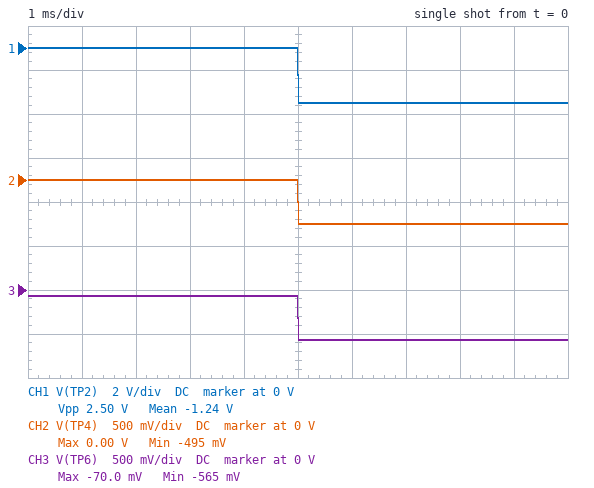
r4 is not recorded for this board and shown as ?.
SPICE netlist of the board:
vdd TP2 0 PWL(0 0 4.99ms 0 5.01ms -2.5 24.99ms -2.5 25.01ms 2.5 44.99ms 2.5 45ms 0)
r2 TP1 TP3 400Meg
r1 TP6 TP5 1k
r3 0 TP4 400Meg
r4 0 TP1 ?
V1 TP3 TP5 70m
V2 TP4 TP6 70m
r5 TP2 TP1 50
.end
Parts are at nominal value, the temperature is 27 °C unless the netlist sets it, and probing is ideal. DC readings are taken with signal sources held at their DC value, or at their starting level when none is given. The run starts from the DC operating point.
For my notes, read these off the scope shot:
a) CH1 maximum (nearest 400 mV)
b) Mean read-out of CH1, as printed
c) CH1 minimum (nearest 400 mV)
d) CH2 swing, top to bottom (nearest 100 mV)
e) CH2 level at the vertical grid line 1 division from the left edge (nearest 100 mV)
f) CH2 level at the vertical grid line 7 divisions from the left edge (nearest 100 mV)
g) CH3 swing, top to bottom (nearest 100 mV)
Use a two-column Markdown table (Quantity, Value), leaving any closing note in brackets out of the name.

| Quantity | Value |
|---|---|
| CH1 maximum | 0 V |
| Mean read-out of CH1, as printed | -1.24 V |
| CH1 minimum | -2.4 V |
| CH2 swing, top to bottom | 500 mV |
| CH2 level at the vertical grid line 1 division from the left edge | 0 V |
| CH2 level at the vertical grid line 7 divisions from the left edge | -500 mV |
| CH3 swing, top to bottom | 500 mV |
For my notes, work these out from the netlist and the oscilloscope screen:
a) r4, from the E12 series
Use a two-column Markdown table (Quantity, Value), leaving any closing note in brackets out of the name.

| Quantity | Value |
|---|---|
| r4, from the E12 series | 33 Ω |
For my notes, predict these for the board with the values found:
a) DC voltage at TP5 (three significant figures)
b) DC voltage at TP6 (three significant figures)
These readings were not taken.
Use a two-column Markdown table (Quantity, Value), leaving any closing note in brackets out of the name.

| Quantity | Value |
|---|---|
| DC voltage at TP5 | -70.0 mV |
| DC voltage at TP6 | -70.0 mV |
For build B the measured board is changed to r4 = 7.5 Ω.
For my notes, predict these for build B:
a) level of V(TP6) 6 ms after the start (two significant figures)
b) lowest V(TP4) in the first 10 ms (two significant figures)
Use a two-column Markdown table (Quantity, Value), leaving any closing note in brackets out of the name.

| Quantity | Value |
|---|---|
| level of V(TP6) 6 ms after the start | -230 mV |
| lowest V(TP4) in the first 10 ms | -160 mV |
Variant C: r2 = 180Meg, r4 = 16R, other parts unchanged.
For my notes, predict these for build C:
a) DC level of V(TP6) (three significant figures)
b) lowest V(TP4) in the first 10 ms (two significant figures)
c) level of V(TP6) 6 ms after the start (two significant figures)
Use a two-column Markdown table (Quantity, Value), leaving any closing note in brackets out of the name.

| Quantity | Value |
|---|---|
| DC level of V(TP6) | -70.0 mV |
| lowest V(TP4) in the first 10 ms | -420 mV |
| level of V(TP6) 6 ms after the start | -490 mV |
